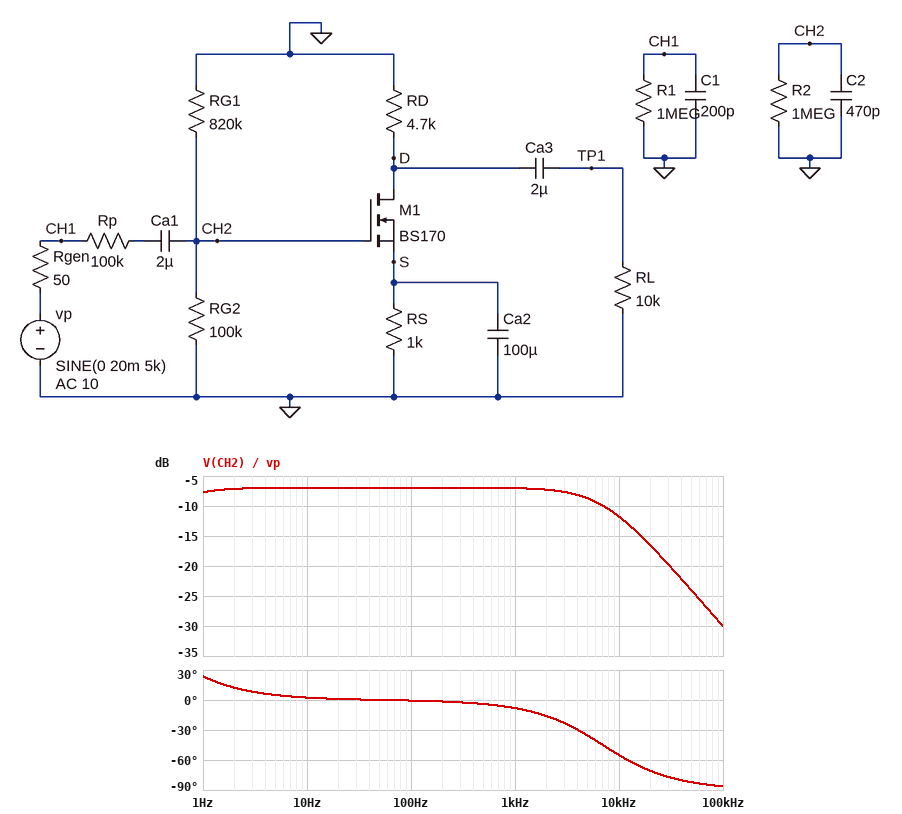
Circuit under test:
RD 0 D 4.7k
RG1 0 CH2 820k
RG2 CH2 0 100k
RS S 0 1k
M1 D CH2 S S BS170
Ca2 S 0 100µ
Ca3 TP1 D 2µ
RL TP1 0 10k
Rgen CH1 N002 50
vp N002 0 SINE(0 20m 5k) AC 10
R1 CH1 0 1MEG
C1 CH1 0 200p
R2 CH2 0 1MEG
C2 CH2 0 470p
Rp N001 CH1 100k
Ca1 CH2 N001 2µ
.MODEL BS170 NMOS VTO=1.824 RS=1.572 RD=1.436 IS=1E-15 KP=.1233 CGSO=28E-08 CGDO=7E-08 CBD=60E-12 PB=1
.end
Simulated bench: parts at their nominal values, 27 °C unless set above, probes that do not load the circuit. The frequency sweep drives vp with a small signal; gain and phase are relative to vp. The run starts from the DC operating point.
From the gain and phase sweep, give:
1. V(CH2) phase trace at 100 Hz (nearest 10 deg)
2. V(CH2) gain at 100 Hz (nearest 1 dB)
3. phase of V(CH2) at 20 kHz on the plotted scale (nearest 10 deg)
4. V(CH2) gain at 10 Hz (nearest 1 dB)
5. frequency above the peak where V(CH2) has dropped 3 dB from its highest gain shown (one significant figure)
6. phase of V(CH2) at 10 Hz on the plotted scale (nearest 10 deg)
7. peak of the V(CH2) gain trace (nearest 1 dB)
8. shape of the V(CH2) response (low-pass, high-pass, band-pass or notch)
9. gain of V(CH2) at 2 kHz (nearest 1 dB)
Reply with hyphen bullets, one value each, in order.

- 0 deg
- -7 dB
- -70 deg
- -7 dB
- 7 kHz
- 0 deg
- -7 dB
- low-pass
- -7 dB
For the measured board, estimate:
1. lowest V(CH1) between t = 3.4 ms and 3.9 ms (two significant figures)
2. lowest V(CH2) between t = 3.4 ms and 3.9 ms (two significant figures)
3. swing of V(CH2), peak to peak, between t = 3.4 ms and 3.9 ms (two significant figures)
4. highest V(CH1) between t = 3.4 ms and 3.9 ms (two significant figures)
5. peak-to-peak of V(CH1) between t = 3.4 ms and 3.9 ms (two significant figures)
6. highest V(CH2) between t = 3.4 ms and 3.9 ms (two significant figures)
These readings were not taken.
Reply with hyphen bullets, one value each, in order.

- -20 mV
- -7.3 mV
- 15 mV
- 20 mV
- 40 mV
- 7.3 mV
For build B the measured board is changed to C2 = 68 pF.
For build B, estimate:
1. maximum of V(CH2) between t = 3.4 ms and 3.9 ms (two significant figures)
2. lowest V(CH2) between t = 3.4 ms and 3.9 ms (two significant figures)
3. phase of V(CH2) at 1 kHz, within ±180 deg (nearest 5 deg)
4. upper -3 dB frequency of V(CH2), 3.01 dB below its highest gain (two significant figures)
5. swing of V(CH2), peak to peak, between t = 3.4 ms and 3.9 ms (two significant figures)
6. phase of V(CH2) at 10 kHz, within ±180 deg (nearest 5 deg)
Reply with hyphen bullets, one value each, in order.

- 8.9 mV
- -8.9 mV
- 0 deg
- 34 kHz
- 18 mV
- -15 deg
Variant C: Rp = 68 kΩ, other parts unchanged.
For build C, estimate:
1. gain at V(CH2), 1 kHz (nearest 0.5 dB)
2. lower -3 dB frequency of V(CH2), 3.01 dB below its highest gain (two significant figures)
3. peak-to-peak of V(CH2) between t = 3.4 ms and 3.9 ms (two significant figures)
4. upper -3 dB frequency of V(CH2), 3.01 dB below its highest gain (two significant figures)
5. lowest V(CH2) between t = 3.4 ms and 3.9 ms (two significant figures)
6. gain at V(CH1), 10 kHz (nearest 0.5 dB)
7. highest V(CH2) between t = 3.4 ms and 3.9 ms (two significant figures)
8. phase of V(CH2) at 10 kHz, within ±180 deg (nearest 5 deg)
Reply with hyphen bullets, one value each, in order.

- -5.5 dB
- 530 mHz
- 19 mV
- 8.5 kHz
- -9.4 mV
- 0 dB
- 9.4 mV
- -50 deg
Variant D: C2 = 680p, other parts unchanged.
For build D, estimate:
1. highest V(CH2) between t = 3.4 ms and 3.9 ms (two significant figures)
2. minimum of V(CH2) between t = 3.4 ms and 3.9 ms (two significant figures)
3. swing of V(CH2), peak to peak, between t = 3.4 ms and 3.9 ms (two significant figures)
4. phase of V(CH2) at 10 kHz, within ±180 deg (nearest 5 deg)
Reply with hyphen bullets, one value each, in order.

- 6.3 mV
- -6.3 mV
- 13 mV
- -65 deg
